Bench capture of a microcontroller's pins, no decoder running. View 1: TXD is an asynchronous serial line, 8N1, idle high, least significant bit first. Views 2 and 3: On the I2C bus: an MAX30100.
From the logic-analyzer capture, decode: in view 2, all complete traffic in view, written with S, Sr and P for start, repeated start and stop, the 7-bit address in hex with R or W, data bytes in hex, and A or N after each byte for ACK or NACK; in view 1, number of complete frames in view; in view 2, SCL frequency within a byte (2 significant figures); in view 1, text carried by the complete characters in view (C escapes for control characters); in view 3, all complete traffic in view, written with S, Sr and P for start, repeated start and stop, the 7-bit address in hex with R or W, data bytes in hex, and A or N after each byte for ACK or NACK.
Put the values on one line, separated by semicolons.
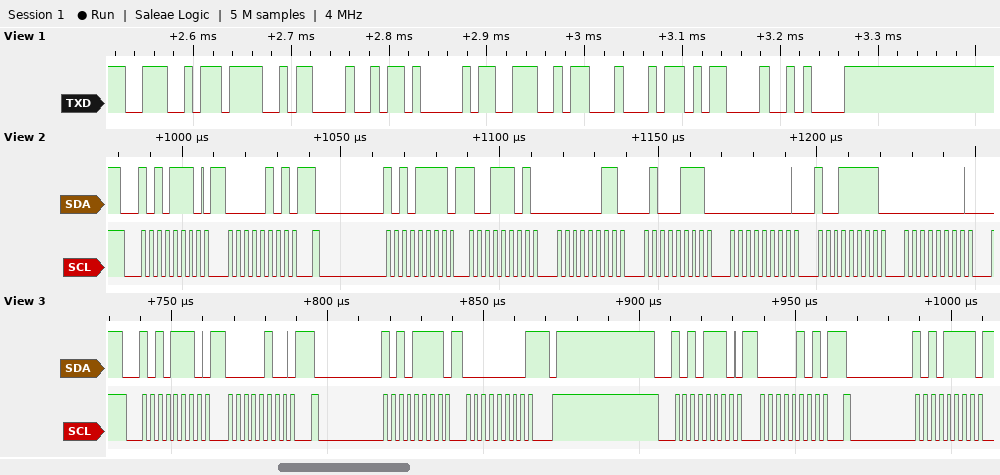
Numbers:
S 57W A 05 A Sr 57R A 9D A 03 A 47 A 00 A 9F A 00 A; 8; 400 kHz; "NOHAND\r\n"; S 57W A 04 A Sr 57R A 00 N P S 57W A 05 A Sr 57R A
